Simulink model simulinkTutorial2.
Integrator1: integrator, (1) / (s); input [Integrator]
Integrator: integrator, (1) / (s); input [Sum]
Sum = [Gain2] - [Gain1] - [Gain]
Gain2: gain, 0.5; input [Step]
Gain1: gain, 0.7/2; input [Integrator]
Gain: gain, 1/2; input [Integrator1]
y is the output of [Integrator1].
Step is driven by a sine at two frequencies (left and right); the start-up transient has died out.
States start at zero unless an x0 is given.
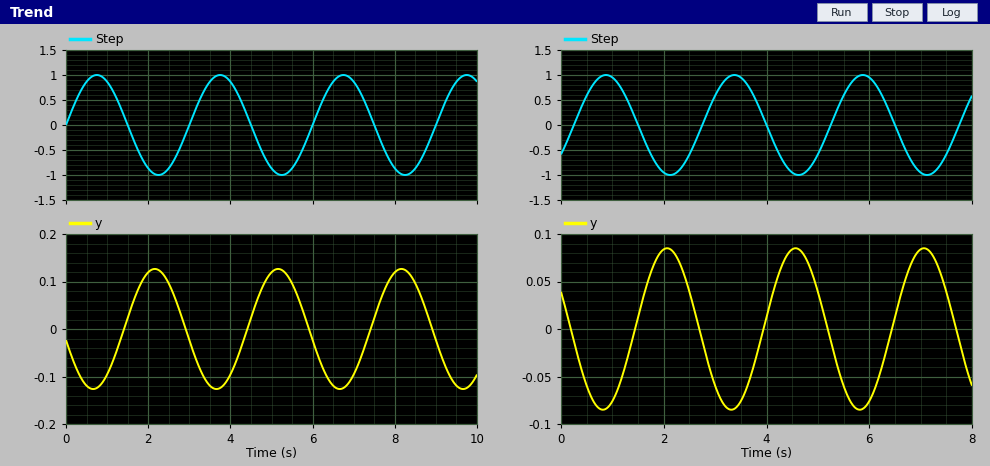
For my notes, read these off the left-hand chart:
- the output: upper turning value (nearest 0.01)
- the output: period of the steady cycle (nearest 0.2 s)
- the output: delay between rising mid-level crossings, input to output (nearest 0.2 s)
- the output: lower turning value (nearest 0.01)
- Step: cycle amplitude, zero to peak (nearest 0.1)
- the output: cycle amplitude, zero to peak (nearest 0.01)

0.13
3.0 s
1.4 s
-0.13
1.0
0.13
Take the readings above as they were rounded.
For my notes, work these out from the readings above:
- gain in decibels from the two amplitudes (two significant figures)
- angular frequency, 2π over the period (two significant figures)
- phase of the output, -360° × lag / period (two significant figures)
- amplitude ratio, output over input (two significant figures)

-18 dB
2.1 rad/s
-170°
0.13
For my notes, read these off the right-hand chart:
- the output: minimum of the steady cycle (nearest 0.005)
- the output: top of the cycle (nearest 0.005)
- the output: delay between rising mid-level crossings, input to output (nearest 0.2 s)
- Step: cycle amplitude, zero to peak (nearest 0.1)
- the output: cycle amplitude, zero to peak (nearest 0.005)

-0.085
0.085
1.2 s
1.0
0.085
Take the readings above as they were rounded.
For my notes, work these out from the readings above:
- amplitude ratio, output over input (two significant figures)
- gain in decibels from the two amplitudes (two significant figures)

0.085
-21 dB
